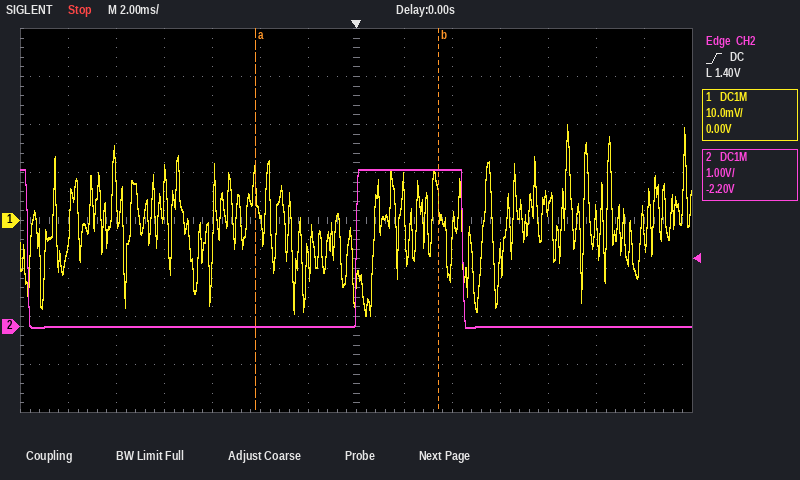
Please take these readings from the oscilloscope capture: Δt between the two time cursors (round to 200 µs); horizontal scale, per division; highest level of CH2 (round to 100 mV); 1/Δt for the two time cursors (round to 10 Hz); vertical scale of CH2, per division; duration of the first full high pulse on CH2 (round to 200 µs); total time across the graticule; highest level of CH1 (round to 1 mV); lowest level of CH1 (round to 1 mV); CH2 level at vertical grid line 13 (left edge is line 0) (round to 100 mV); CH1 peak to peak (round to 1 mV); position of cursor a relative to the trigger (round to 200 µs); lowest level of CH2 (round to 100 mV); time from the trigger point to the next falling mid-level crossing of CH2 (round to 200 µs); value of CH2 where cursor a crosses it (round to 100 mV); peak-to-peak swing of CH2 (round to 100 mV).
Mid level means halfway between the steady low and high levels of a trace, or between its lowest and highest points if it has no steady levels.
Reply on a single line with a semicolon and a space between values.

7.6 ms; 2 ms; 3.3 V; 130 Hz; 1 V; 4.4 ms; 28 ms; 20 mV; -20 mV; 0.0 V; 40 mV; -4.2 ms; 0.0 V; 4.4 ms; 0.0 V; 3.3 V
